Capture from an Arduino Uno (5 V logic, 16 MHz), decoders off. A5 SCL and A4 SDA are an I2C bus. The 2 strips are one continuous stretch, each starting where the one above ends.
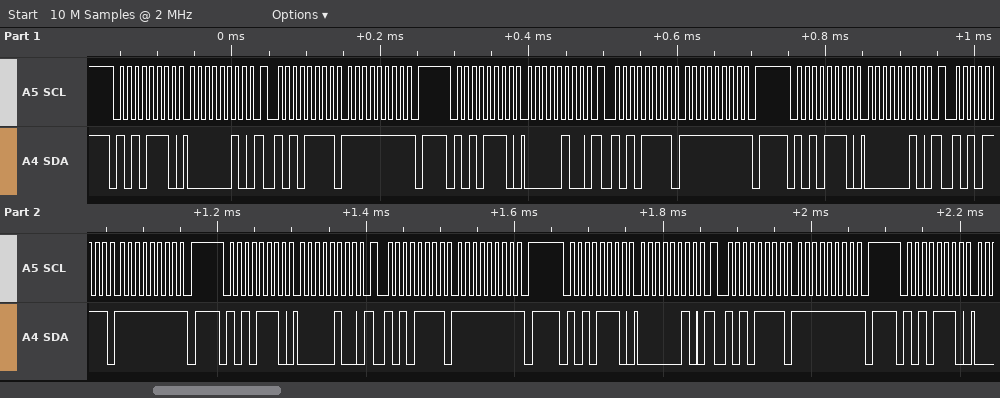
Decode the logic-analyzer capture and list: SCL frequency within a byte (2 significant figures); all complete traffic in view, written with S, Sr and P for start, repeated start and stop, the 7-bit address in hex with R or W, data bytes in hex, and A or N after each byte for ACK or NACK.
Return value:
100 kHz
S 57W A 02 A Sr 57R A FF N P S 57W A 04 A Sr 57R A FF N P S 57W A 02 A Sr 57R A FF N P S 57W A 04 A Sr 57R A FF N P S 57W A 02 A Sr 57R A FF N P S 57W A
